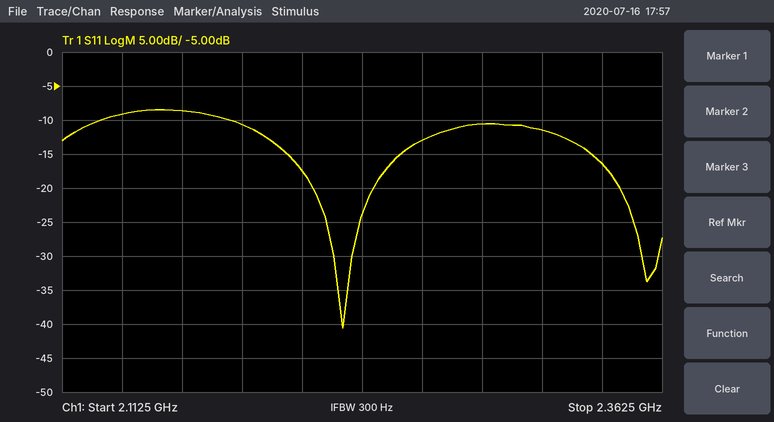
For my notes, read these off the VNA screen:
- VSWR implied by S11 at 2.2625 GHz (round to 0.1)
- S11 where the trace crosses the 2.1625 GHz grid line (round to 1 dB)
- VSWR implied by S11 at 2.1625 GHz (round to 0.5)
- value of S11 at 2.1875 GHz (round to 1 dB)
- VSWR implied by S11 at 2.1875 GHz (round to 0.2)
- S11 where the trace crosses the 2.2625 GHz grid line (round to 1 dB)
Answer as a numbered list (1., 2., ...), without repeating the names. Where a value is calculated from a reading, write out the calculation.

1. |Γ| = 10^(-13/20) = 0.2239; VSWR = (1 + 0.2239)/(1 − 0.2239) ≈ 1.6
2. -9 dB
3. |Γ| = 10^(-9/20) = 0.3548; VSWR = (1 + 0.3548)/(1 − 0.3548) ≈ 2.10, so 2.0 to the nearest 0.5
4. -11 dB
5. |Γ| = 10^(-11/20) = 0.2818; VSWR = (1 + 0.2818)/(1 − 0.2818) ≈ 1.8
6. -13 dB
